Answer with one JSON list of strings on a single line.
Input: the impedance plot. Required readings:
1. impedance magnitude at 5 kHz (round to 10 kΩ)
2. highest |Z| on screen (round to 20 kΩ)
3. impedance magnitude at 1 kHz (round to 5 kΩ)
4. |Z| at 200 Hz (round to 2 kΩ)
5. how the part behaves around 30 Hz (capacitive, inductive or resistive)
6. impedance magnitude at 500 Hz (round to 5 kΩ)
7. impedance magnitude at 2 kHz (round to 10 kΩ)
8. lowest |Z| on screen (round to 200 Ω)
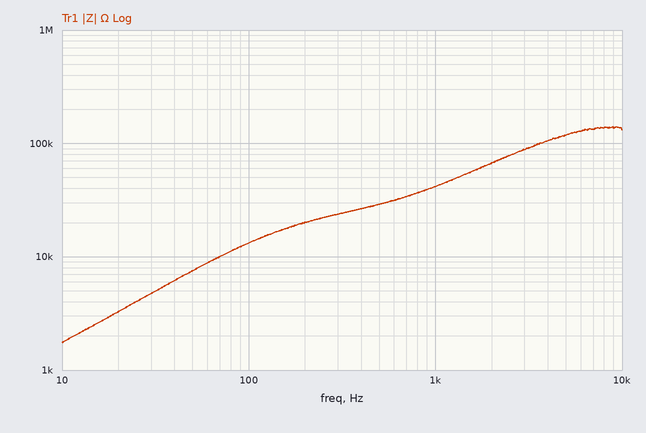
["120 kΩ", "140 kΩ", "40 kΩ", "20 kΩ", "inductive", "30 kΩ", "70 kΩ", "1.8 kΩ"]
